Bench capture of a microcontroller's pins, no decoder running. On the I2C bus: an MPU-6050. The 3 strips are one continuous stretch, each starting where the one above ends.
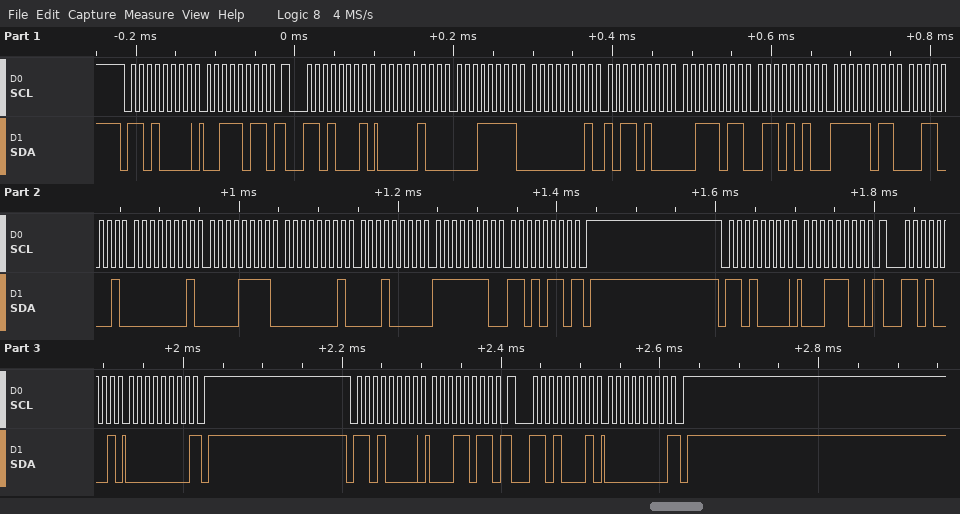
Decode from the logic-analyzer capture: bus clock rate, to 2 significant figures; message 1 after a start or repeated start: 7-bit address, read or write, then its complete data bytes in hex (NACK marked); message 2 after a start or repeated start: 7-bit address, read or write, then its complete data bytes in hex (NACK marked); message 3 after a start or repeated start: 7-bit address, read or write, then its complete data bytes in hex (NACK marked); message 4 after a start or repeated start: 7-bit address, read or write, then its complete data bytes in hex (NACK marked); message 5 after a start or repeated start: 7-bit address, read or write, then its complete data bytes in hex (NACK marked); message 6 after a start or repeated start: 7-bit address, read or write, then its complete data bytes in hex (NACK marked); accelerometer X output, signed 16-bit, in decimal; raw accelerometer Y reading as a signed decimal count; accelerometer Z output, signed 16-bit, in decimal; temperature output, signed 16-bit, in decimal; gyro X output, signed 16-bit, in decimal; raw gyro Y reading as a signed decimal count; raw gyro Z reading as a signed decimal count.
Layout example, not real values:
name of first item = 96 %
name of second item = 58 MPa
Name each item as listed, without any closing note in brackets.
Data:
bus clock rate, to 2 significant figures = 100 kHz
message 1 after a start or repeated start: 7-bit address, read or write, then its complete data bytes in hex = 0x68 write: 3B
message 2 after a start or repeated start: 7-bit address, read or write, then its complete data bytes in hex = 0x68 read: 04 1F 01 B4 3B 6A FB 31 01 0F 01 10 FE D6 NACK
message 3 after a start or repeated start: 7-bit address, read or write, then its complete data bytes in hex = 0x68 write: 1C
message 4 after a start or repeated start: 7-bit address, read or write, then its complete data bytes in hex = 0x68 read: 00 NACK
message 5 after a start or repeated start: 7-bit address, read or write, then its complete data bytes in hex = 0x68 write: 1B
message 6 after a start or repeated start: 7-bit address, read or write, then its complete data bytes in hex = 0x68 read: 00 NACK
accelerometer X output, signed 16-bit, in decimal = 1055
raw accelerometer Y reading as a signed decimal count = 436
accelerometer Z output, signed 16-bit, in decimal = 15210
temperature output, signed 16-bit, in decimal = -1231
gyro X output, signed 16-bit, in decimal = 271
raw gyro Y reading as a signed decimal count = 272
raw gyro Z reading as a signed decimal count = -298
